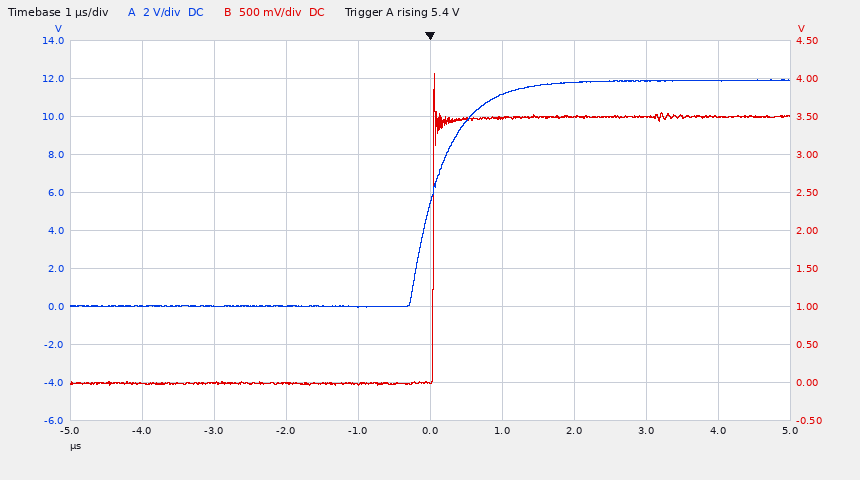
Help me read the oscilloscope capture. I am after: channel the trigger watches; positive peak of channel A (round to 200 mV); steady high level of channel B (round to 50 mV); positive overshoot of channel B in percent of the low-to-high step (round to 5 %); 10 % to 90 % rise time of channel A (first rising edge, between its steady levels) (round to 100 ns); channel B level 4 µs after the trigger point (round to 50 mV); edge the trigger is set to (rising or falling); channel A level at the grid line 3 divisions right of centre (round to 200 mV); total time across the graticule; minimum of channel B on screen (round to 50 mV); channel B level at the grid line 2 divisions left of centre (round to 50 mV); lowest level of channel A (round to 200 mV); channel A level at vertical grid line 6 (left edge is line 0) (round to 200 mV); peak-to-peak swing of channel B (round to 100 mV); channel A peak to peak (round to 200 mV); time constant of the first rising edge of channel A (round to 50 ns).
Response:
channel A
12.0 V
3.50 V
15 %
1.0 µs
3.50 V
rising
11.8 V
10 µs
-50 mV
0 mV
0.0 V
11.2 V
4.10 V
12.0 V
450 ns
